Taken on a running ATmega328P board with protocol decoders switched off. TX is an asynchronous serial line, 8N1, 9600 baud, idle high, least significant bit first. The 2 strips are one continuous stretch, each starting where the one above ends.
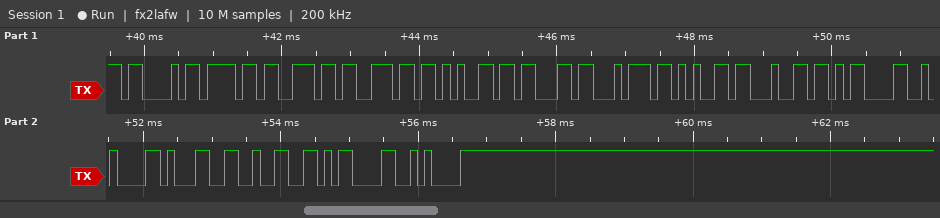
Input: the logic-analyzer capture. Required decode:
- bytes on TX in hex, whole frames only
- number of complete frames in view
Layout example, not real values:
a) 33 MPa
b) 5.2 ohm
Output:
a) 0x43 0x6F 0x6E 0x6E 0x65 0x63 0x74 0x65 0x64 0x0D 0x0A 0x31 0x32 0x0D 0x0A
b) 15
